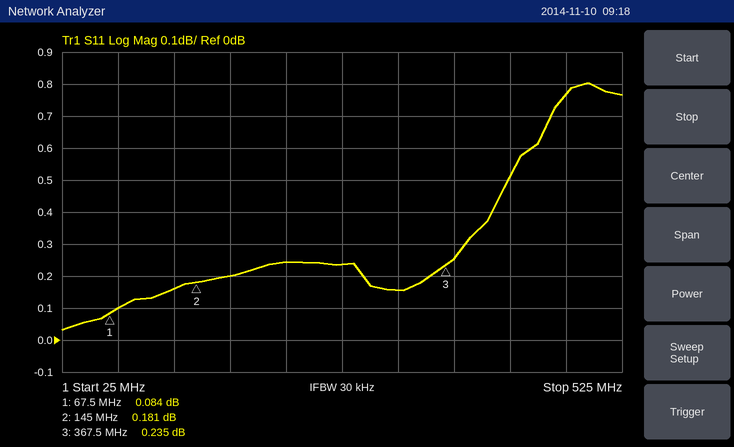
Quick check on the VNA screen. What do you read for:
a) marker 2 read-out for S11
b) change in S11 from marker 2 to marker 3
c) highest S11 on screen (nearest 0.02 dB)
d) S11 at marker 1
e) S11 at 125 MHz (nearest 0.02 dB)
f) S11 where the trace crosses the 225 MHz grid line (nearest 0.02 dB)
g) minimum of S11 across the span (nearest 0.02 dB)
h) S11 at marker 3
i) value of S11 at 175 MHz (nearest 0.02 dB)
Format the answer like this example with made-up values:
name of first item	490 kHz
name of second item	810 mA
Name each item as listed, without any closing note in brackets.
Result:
marker 2 read-out for S11	0.181 dB
change in S11 from marker 2 to marker 3	0.054 dB
highest S11 on screen	0.80 dB
S11 at marker 1	0.084 dB
S11 at 125 MHz	0.16 dB
S11 where the trace crosses the 225 MHz grid line	0.24 dB
minimum of S11 across the span	0.04 dB
S11 at marker 3	0.235 dB
value of S11 at 175 MHz	0.20 dB
